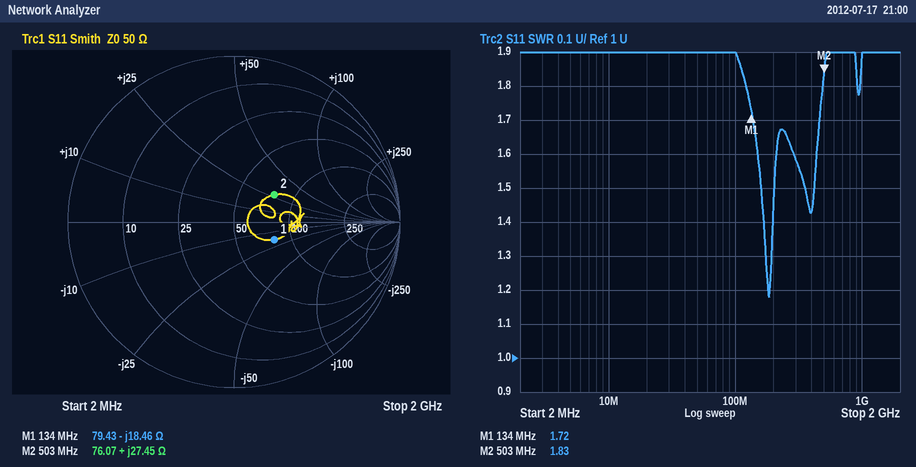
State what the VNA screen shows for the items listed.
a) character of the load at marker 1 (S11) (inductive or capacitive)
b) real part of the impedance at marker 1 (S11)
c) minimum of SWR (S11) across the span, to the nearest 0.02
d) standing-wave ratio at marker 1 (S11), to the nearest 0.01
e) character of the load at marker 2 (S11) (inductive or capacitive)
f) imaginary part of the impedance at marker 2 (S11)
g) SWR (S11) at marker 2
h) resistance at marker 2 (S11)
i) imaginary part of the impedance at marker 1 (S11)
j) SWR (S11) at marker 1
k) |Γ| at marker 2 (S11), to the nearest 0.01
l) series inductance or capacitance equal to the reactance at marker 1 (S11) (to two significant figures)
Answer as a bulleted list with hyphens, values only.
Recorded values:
- capacitive
- 79.43 Ω
- 1.18
- 1.72
- inductive
- +27.45 Ω
- 1.83
- 76.07 Ω
- -18.46 Ω
- 1.72
- 0.29
- 64 pF
